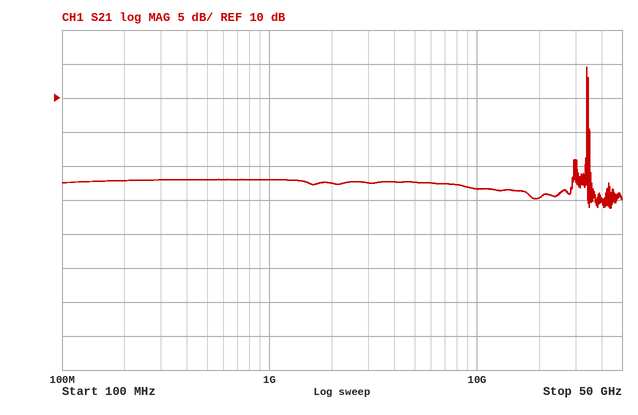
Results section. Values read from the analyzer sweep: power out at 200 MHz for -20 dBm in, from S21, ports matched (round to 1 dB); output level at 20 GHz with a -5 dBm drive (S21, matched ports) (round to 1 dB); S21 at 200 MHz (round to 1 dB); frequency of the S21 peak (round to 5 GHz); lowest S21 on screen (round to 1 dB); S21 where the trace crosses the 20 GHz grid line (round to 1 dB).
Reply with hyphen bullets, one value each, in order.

- -22 dBm
- -10 dBm
- -2 dB
- 35 GHz
- -6 dB
- -5 dB
